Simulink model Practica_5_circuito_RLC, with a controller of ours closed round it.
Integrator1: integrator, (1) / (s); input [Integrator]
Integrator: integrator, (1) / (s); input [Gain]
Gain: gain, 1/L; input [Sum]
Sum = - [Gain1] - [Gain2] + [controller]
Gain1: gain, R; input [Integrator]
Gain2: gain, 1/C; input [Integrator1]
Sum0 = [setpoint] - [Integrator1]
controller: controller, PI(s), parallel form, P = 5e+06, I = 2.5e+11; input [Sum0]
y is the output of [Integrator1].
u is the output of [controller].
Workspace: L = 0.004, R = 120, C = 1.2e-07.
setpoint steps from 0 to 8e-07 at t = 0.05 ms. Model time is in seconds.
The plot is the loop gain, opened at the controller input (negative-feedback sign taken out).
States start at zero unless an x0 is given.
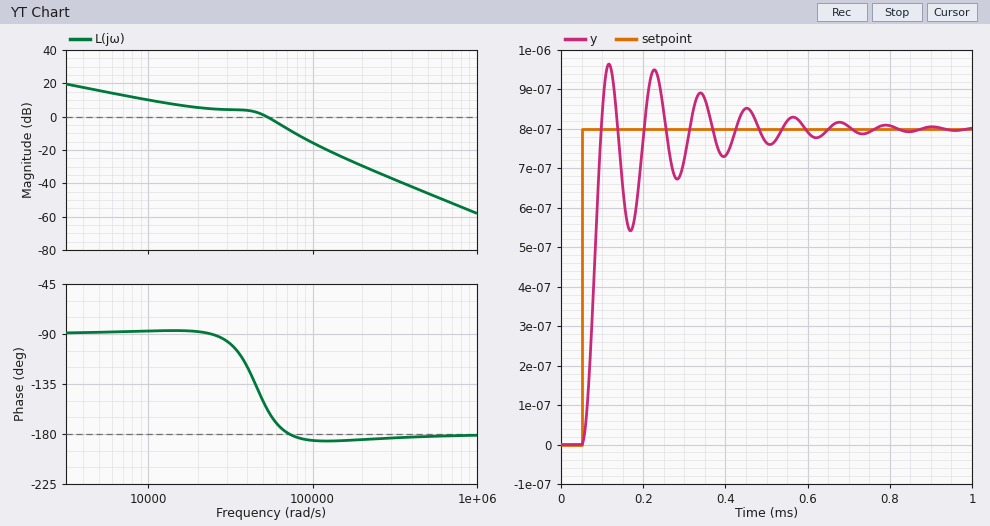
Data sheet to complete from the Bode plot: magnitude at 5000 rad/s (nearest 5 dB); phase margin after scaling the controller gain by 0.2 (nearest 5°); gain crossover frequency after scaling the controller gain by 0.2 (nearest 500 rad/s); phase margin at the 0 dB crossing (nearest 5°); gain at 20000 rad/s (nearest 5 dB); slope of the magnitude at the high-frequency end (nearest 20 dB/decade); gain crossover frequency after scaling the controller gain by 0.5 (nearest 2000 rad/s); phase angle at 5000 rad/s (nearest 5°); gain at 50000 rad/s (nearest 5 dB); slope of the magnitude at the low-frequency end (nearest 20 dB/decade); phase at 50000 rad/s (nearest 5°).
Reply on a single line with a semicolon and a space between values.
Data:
15 dB; 90°; 6000 rad/s; 25°; 5 dB; -40 dB/decade; 18000 rad/s; -90°; 0 dB; -20 dB/decade; -150°
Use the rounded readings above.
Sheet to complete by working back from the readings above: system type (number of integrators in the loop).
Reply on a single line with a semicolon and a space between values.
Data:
1
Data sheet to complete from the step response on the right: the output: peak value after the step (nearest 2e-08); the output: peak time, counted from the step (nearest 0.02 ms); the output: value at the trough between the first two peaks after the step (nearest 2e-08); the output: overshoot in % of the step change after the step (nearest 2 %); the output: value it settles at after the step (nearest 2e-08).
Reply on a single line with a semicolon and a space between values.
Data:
0.00000096; 0.06 ms; 0.00000054; 20 %; 0.00000080
